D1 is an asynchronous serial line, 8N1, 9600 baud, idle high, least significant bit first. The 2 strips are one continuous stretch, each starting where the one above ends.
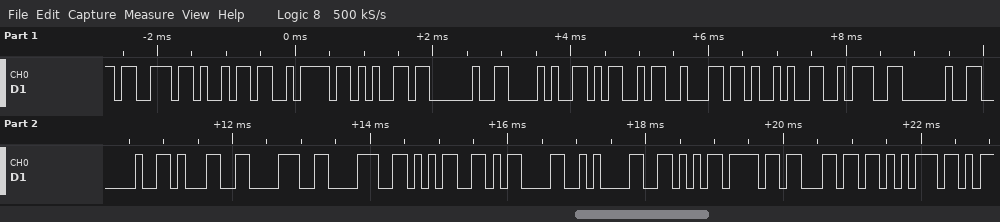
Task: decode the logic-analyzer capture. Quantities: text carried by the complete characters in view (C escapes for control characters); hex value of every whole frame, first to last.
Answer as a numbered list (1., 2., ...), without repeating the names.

1. "size (Mb):  1885\r\nVolu"
2. 73 69 7A 65 20 28 4D 62 29 3A 20 20 31 38 38 35 0D 0A 56 6F 6C 75
